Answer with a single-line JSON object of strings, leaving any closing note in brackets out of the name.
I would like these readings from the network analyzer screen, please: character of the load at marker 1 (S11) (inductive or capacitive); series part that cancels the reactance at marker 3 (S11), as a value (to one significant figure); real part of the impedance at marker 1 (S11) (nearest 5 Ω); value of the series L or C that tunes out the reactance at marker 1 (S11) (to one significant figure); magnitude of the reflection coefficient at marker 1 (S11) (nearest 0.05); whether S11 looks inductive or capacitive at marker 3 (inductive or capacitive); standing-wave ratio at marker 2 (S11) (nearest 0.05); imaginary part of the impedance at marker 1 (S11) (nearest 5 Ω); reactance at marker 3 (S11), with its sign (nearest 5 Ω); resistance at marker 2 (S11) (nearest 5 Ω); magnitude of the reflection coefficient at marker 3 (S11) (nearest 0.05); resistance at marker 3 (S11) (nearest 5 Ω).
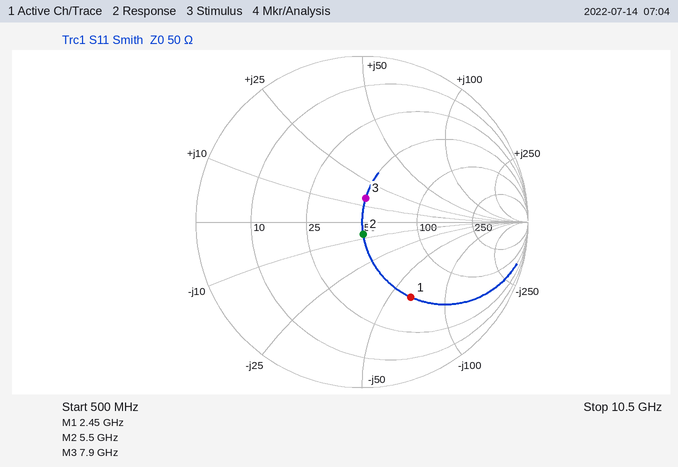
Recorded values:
{"character of the load at marker 1 (S11)": "capacitive", "series part that cancels the reactance at marker 3 (S11), as a value": "1 pF", "real part of the impedance at marker 1 (S11)": "50 Ω", "value of the series L or C that tunes out the reactance at marker 1 (S11)": "4 nH", "magnitude of the reflection coefficient at marker 1 (S11)": "0.55", "whether S11 looks inductive or capacitive at marker 3": "inductive", "standing-wave ratio at marker 2 (S11)": "1.15", "imaginary part of the impedance at marker 1 (S11)": "-65 Ω", "reactance at marker 3 (S11), with its sign": "+15 Ω", "resistance at marker 2 (S11)": "50 Ω", "magnitude of the reflection coefficient at marker 3 (S11)": "0.15", "resistance at marker 3 (S11)": "50 Ω"}
